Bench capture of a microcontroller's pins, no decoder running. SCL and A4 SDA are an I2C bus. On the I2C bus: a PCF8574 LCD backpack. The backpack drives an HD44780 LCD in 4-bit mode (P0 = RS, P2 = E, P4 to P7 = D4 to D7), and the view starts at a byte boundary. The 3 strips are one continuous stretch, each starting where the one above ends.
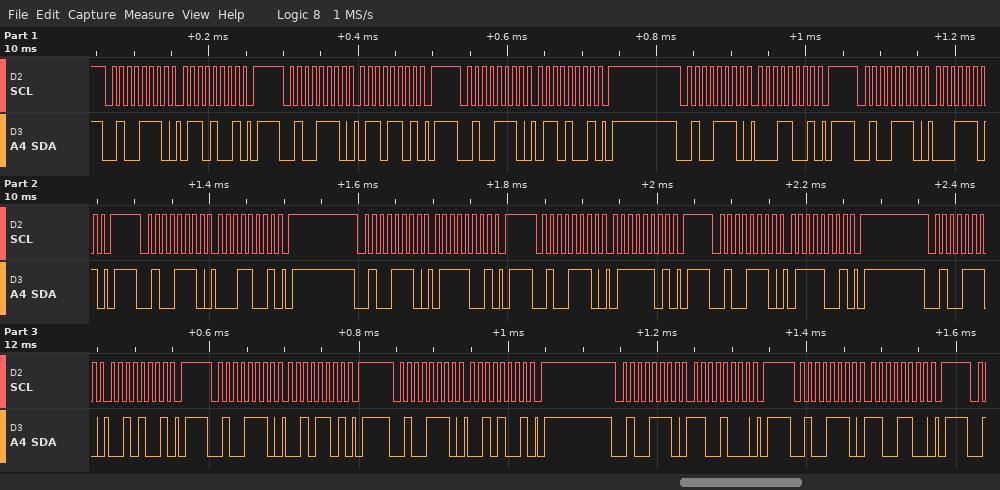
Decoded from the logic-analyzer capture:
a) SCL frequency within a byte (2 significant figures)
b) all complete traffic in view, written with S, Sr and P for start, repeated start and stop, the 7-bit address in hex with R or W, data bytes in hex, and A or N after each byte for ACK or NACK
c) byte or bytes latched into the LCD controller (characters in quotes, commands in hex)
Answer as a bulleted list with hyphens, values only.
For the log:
- 100 kHz
- S 27W A 69 A P S 27W A 6D A P S 27W A 69 A P S 27W A 19 A P S 27W A 1D A P S 27W A 19 A P S 27W A 79 A P S 27W A 7D A P S 27W A 79 A P S 27W A 29 A P S 27W A 2D A P S 27W A 29 A P S 27W A C8 A P S 27W A CC A P
- 'a' 'r'
